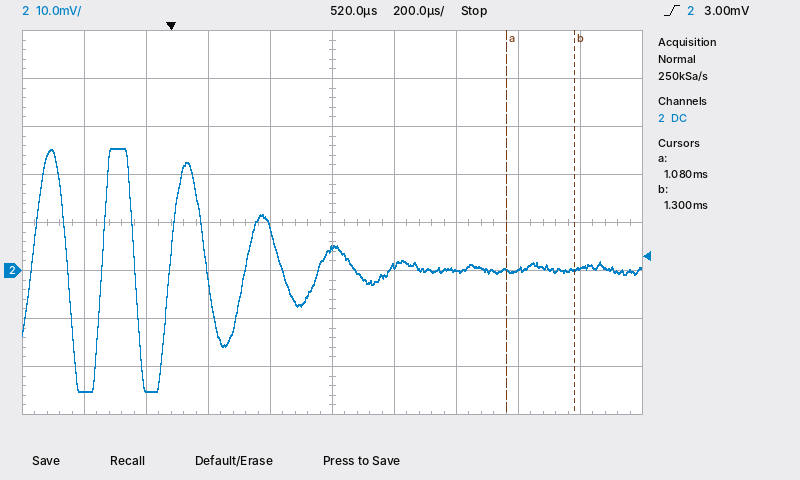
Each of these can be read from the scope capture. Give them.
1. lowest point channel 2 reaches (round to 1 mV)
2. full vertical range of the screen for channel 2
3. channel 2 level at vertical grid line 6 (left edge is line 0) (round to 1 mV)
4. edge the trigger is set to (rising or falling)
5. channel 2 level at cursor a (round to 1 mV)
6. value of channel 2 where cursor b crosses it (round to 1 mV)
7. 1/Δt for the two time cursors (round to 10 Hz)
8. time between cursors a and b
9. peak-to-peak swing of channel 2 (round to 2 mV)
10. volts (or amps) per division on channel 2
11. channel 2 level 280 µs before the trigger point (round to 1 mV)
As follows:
-25 mV
80 mV
1 mV
rising
0 mV
0 mV
4.55 kHz
220 µs
50 mV
10 mV
-25 mV
